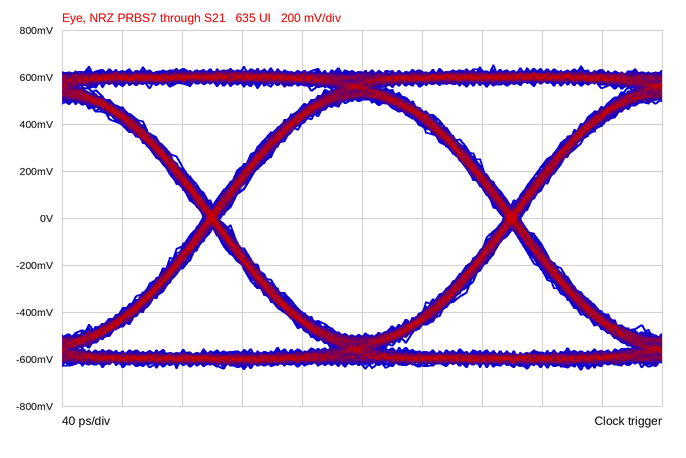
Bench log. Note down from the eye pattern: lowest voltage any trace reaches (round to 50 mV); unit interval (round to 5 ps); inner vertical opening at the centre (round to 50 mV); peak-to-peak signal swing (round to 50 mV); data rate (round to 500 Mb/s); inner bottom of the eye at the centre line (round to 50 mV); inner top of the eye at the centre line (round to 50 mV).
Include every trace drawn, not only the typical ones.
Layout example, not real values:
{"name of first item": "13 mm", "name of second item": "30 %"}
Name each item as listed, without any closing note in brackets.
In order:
{"lowest voltage any trace reaches": "-650 mV", "unit interval": "200 ps", "inner vertical opening at the centre": "1.00 V", "peak-to-peak signal swing": "1.30 V", "data rate": "5.0 Gb/s", "inner bottom of the eye at the centre line": "-500 mV", "inner top of the eye at the centre line": "500 mV"}
